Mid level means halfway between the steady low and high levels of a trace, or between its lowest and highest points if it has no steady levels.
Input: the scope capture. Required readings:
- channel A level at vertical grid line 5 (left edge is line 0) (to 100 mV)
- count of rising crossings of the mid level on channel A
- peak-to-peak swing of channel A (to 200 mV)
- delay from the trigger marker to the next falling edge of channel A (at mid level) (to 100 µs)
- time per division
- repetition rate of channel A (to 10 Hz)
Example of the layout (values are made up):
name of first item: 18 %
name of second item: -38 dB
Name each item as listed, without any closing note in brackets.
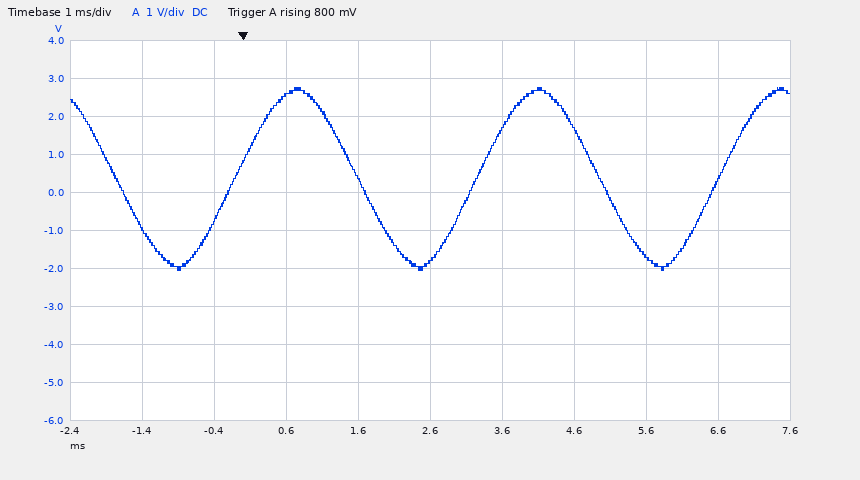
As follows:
channel A level at vertical grid line 5 (left edge is line 0): -1.8 V
count of rising crossings of the mid level on channel A: 3
peak-to-peak swing of channel A: 4.8 V
delay from the trigger marker to the next falling edge of channel A (at mid level): 1.6 ms
time per division: 1 ms
repetition rate of channel A: 300 Hz
